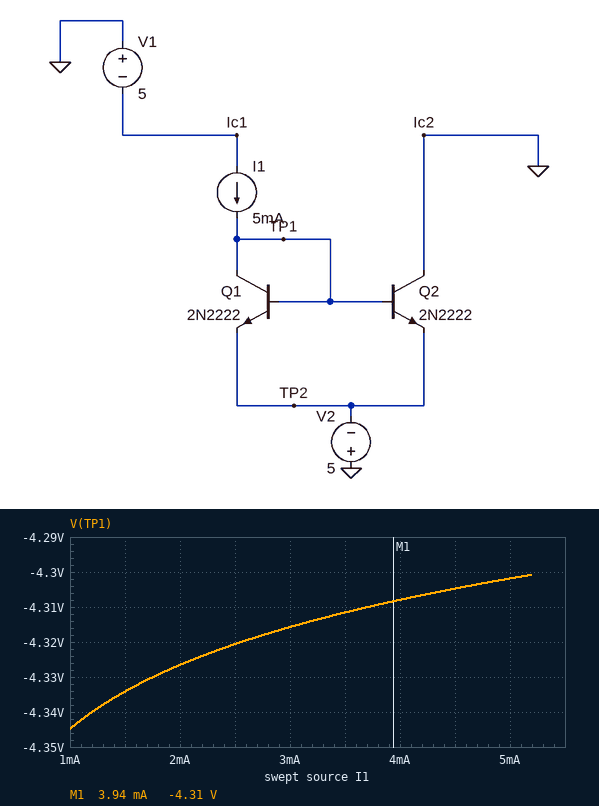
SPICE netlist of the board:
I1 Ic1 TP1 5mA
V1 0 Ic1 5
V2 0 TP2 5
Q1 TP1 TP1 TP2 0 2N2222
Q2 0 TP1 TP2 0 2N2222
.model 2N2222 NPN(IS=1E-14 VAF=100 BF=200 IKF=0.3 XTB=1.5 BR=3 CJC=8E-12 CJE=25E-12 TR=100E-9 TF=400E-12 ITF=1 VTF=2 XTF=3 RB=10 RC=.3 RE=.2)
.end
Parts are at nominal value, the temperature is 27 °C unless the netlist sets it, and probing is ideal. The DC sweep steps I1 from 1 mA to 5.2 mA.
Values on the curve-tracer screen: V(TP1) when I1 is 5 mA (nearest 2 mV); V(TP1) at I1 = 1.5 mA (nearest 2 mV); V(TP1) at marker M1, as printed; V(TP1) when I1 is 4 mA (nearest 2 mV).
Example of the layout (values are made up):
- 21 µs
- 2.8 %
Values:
- -4.302 V
- -4.334 V
- -4.31 V
- -4.308 V
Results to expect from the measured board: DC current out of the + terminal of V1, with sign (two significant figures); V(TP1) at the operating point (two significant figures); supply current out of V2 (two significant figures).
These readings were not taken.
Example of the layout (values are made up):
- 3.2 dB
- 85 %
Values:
- -5.0 mA
- -4.3 V
- 10 mA
